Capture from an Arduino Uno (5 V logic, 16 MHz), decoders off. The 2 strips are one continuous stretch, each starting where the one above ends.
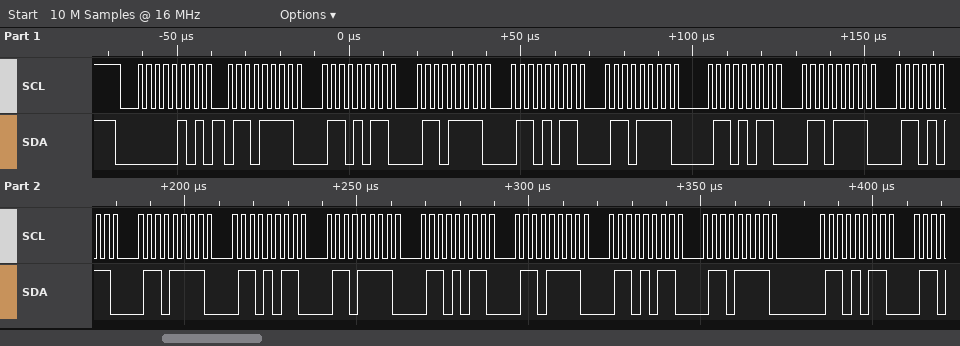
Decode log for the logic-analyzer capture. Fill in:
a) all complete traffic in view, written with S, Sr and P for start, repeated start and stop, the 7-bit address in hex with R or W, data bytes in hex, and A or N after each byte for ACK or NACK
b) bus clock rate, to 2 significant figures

S 02R A 6F A 6B A 6F A 6B A 6F A 6B A 6F A 6B A 6F A 6B A 6F A 6B A 6F A 6B A 6F A 6B A
400 kHz
